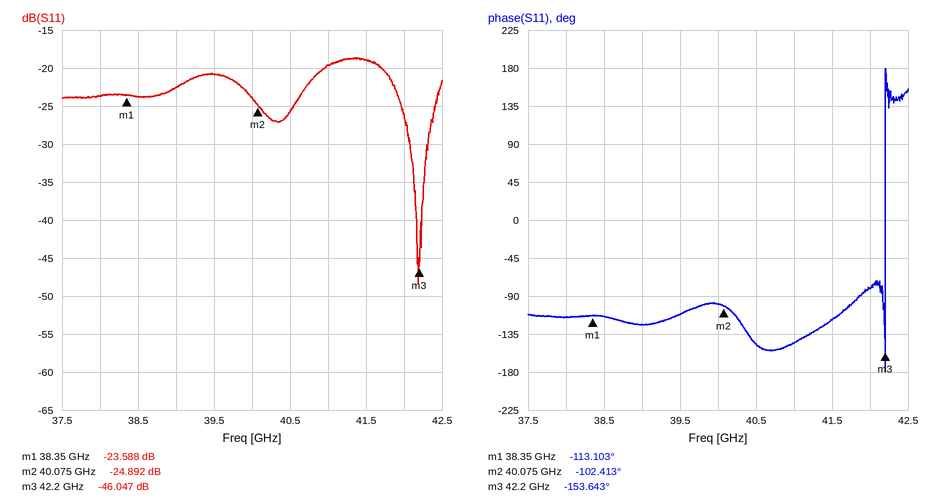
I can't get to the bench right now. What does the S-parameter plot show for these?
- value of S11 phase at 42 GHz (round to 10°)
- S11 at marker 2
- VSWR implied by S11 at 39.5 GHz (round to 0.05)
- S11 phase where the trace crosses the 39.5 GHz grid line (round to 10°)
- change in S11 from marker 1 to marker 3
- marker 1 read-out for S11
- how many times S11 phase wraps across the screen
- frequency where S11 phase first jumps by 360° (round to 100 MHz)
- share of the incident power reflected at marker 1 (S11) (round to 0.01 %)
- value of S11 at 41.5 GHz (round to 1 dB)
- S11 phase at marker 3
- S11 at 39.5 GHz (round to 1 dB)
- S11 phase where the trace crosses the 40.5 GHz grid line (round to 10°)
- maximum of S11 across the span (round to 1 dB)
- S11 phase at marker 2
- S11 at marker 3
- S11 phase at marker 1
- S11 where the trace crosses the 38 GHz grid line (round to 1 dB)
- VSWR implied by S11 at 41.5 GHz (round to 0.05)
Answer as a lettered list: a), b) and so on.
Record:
a) -80°
b) -24.892 dB
c) 1.20
d) -110°
e) -22.459 dB
f) -23.588 dB
g) 1
h) 42.2 GHz
i) 0.44 %
j) -19 dB
k) -153.643°
l) -21 dB
m) -150°
n) -19 dB
o) -102.413°
p) -46.047 dB
q) -113.103°
r) -24 dB
s) 1.25
